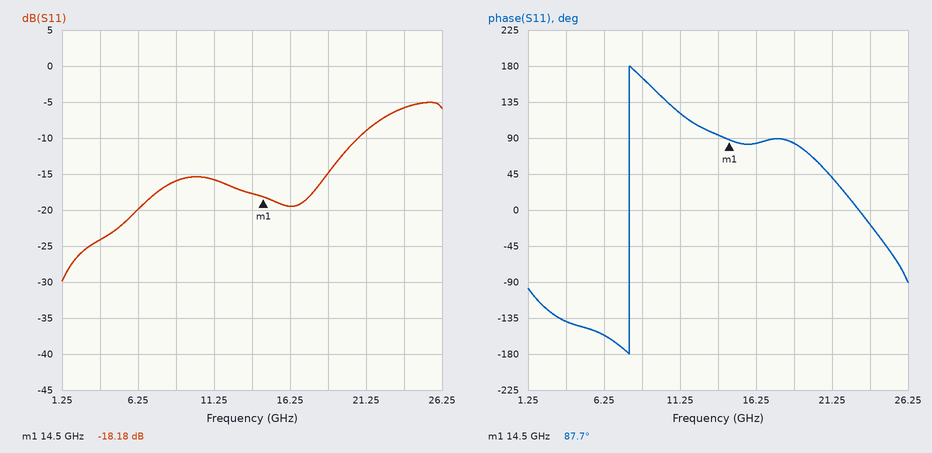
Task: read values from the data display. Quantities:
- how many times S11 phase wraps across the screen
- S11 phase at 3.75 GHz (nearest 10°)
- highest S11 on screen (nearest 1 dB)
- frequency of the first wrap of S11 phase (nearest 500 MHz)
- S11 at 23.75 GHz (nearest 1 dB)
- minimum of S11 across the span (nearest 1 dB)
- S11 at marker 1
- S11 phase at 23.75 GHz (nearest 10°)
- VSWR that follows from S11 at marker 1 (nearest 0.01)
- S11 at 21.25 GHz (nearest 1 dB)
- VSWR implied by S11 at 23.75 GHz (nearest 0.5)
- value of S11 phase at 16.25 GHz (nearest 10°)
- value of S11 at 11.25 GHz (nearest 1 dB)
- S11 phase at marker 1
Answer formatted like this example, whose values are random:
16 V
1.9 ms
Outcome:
1
-140°
-5 dB
8.0 GHz
-6 dB
-30 dB
-18.18 dB
-20°
1.28
-9 dB
3.0
80°
-16 dB
87.7°
